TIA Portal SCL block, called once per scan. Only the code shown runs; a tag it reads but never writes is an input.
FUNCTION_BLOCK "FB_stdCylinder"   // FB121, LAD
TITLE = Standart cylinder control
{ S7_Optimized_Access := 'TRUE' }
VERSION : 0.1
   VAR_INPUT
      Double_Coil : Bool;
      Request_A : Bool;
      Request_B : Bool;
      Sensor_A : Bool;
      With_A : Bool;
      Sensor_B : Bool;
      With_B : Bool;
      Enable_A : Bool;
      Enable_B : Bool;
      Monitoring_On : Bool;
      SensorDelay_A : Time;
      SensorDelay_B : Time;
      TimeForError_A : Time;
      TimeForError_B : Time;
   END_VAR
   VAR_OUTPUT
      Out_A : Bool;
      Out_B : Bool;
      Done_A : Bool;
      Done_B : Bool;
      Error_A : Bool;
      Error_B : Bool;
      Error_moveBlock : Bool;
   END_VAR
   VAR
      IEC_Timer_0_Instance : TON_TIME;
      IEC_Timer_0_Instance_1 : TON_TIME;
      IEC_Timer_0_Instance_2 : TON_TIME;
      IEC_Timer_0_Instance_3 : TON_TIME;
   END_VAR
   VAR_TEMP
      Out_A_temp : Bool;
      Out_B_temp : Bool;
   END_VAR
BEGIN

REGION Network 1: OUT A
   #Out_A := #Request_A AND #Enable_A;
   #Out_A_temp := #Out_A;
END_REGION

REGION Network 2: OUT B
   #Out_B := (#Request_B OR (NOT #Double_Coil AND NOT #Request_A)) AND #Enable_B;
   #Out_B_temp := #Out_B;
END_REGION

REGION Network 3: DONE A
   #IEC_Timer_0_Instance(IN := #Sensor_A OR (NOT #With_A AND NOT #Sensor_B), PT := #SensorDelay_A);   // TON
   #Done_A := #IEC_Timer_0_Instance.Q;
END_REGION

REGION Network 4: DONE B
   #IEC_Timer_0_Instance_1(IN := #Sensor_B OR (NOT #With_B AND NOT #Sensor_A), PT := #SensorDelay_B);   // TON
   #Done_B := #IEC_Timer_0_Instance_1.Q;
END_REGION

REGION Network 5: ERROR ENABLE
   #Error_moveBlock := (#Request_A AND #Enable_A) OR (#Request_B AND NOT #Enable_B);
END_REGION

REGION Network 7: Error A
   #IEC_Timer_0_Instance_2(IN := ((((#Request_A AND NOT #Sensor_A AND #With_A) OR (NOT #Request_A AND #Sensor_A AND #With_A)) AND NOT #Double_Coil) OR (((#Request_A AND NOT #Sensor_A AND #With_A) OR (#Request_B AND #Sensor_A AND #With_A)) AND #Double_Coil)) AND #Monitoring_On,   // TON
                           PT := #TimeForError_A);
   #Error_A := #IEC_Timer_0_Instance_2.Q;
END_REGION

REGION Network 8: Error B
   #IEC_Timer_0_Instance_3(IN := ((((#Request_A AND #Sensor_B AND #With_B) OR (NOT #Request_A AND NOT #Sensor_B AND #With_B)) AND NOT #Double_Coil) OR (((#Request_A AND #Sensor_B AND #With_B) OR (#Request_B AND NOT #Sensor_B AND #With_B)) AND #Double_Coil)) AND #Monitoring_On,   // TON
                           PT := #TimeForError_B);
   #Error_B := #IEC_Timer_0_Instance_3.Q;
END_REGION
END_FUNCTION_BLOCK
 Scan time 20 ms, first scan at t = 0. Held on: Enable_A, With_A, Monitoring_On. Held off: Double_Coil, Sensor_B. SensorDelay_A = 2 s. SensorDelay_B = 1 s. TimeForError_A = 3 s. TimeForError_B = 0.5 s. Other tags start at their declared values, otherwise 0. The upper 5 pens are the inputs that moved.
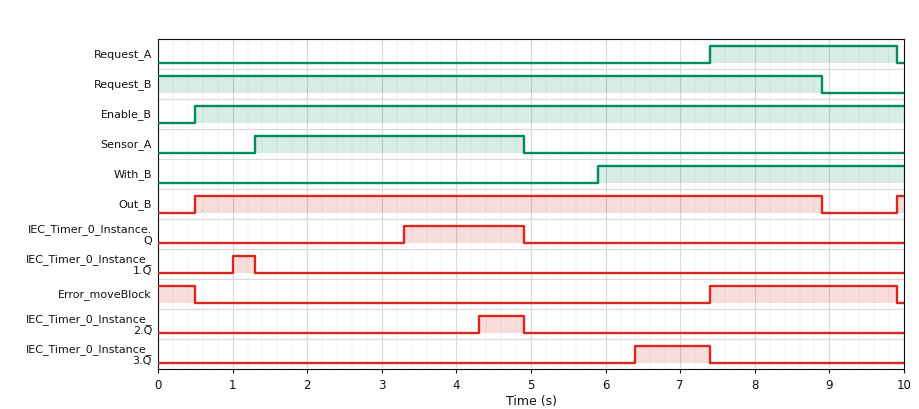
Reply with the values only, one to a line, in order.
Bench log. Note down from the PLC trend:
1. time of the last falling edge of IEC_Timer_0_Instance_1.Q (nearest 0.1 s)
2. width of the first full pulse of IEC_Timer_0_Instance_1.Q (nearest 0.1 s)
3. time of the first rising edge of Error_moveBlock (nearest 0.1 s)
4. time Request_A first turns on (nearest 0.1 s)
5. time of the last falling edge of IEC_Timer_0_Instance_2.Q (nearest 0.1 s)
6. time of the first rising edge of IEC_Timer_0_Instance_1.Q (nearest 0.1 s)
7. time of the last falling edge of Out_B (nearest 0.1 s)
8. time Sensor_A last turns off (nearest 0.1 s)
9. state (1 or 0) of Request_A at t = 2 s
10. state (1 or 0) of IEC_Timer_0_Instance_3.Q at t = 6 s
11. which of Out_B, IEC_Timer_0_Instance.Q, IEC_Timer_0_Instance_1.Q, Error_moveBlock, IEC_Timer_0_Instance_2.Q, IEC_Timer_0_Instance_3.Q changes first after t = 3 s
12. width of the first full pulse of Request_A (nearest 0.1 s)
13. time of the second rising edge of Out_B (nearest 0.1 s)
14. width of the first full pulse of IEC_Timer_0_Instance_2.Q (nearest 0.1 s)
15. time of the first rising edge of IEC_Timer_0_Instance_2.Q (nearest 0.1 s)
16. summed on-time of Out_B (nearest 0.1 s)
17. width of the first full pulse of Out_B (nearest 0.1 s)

1.3 s
0.3 s
7.4 s
7.4 s
4.9 s
1.0 s
8.9 s
4.9 s
0
0
IEC_Timer_0_Instance.Q
2.5 s
9.9 s
0.6 s
4.3 s
8.5 s
8.4 s
